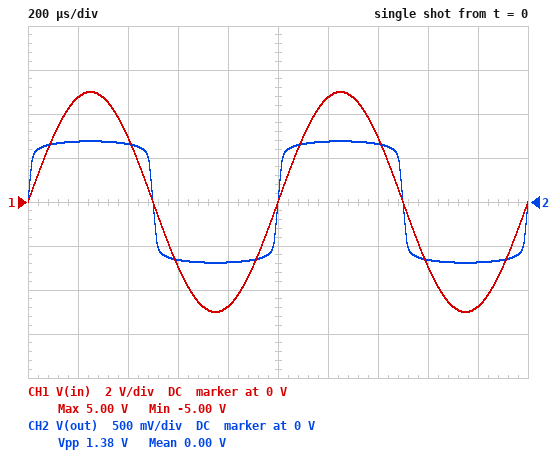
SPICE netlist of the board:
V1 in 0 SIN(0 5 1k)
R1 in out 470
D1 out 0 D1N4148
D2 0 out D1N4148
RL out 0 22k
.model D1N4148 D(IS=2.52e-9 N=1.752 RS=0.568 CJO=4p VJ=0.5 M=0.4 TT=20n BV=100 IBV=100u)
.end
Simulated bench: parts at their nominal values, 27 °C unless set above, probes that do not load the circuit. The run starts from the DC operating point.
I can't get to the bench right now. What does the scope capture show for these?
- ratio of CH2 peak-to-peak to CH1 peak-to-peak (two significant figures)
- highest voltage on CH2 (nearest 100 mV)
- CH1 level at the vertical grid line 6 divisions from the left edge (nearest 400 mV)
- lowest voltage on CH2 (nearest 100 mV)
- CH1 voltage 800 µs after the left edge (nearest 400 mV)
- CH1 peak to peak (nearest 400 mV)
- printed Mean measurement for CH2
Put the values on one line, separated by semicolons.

0.14; 700 mV; 4.8 V; -700 mV; -4.8 V; 10.0 V; 0.00 V
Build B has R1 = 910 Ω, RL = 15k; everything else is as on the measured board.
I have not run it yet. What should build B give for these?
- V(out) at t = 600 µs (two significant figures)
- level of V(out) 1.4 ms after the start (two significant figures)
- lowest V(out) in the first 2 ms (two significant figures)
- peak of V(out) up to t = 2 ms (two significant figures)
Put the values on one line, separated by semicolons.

-630 mV; 630 mV; -660 mV; 660 mV
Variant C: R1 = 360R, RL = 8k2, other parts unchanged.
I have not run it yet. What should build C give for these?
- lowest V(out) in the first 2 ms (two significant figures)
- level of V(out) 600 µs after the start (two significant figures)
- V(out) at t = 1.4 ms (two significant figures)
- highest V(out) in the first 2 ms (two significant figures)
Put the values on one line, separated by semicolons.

-700 mV; -670 mV; 670 mV; 700 mV
